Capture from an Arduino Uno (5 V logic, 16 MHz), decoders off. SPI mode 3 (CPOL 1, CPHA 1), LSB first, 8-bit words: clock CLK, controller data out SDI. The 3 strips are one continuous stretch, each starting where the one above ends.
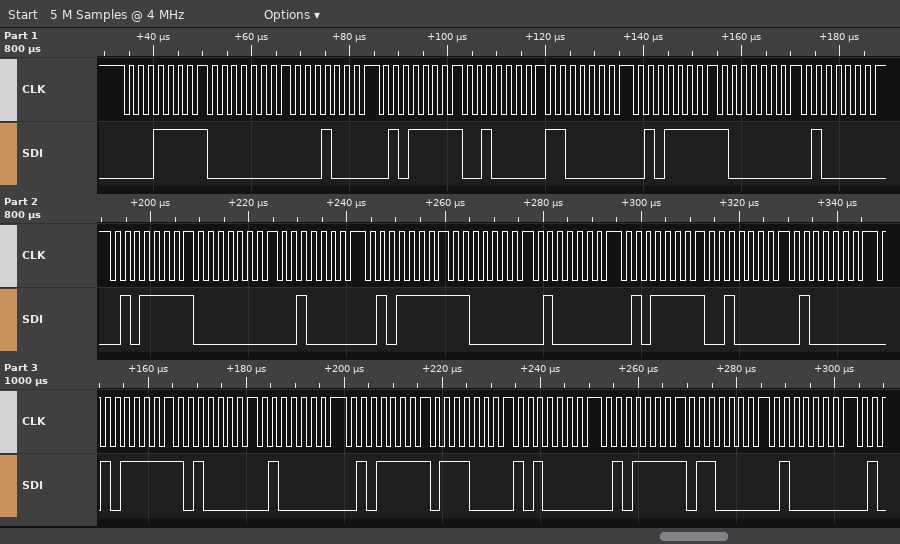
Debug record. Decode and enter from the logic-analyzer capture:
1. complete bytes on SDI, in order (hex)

0xF8 0x00 0x08 0xFA 0x04 0x03 0xFA 0x01 0x02 0xFA 0x00 0x04 0xFA 0x03 0x02 0xFA 0x04 0x02 0xFA 0x05 0x02 0xFA 0x0E 0x05 0xFA 0x06 0x02
